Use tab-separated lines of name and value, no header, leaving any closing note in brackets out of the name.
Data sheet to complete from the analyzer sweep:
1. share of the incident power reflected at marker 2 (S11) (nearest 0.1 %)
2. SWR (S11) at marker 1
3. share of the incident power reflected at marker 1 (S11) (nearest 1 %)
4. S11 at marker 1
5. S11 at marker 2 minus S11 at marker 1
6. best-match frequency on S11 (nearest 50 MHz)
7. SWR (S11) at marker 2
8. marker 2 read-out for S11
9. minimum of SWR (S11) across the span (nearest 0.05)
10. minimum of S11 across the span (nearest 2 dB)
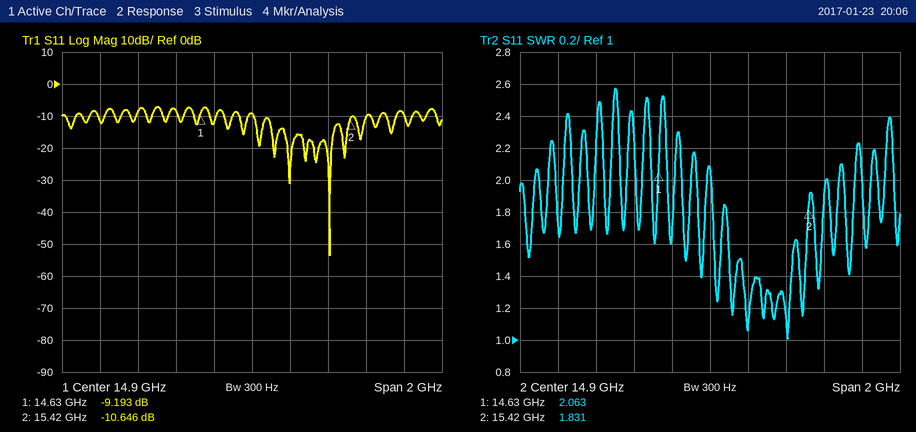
share of the incident power reflected at marker 2 (S11)	8.6 %
SWR (S11) at marker 1	2.063
share of the incident power reflected at marker 1 (S11)	12 %
S11 at marker 1	-9.193 dB
S11 at marker 2 minus S11 at marker 1	-1.453 dB
best-match frequency on S11	15.30 GHz
SWR (S11) at marker 2	1.831
marker 2 read-out for S11	-10.646 dB
minimum of SWR (S11) across the span	1.00
minimum of S11 across the span	-54 dB
